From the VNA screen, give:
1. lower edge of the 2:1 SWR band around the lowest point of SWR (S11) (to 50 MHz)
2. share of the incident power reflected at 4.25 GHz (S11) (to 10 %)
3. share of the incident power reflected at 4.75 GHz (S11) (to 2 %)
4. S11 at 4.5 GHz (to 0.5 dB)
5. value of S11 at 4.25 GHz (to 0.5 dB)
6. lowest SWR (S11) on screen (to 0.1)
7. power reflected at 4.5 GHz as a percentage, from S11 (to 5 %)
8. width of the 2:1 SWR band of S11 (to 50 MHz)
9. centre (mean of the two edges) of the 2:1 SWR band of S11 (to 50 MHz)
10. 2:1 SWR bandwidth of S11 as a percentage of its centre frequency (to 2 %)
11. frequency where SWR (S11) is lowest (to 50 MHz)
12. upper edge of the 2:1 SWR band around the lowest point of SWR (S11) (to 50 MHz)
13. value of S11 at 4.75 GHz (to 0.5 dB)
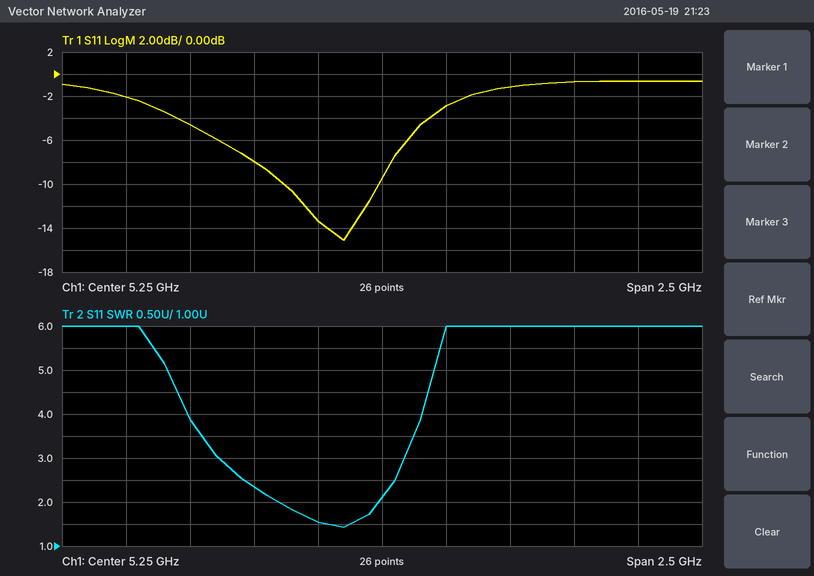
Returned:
4.85 GHz
60 %
16 %
-4.5 dB
-2.0 dB
1.4
35 %
400 MHz
5.05 GHz
8 %
5.10 GHz
5.25 GHz
-8.0 dB
